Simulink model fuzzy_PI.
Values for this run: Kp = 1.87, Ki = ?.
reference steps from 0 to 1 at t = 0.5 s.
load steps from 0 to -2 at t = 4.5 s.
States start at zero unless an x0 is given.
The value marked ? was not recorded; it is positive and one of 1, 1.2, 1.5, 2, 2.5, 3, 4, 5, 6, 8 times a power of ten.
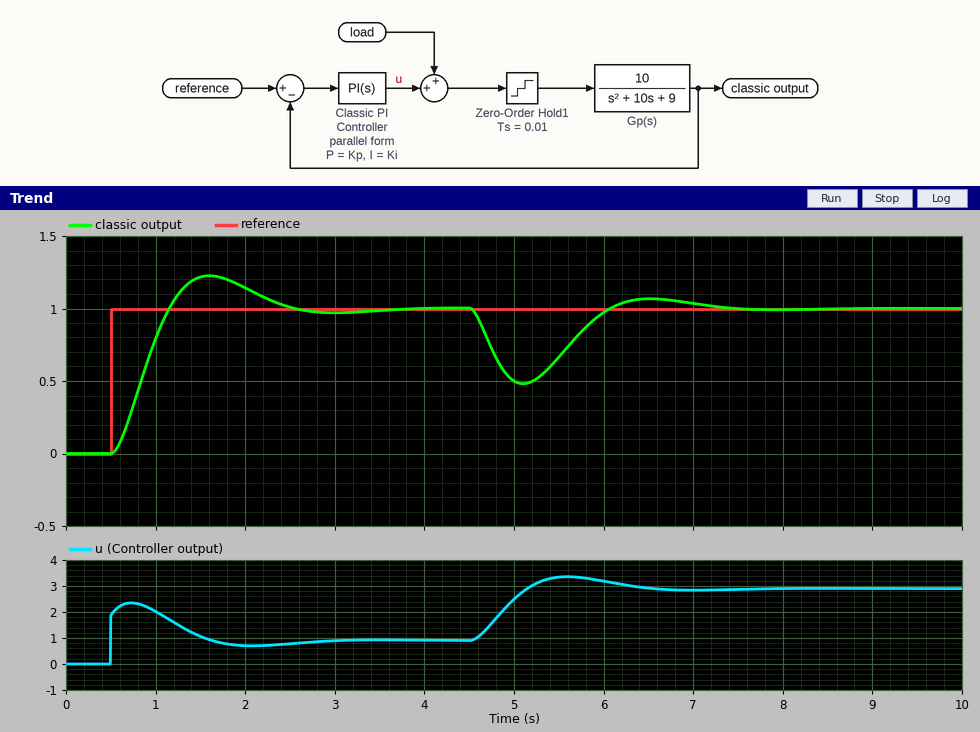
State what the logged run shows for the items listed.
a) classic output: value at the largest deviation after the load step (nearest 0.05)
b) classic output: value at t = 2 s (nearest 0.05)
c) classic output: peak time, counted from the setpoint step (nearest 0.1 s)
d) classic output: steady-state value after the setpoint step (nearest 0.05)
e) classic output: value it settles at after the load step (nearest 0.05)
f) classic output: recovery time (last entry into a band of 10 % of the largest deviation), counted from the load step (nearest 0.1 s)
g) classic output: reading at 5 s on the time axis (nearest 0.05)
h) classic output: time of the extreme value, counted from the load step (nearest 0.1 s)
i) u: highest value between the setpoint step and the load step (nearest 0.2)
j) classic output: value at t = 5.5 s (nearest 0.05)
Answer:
0.50
1.15
1.1 s
1.00
1.00
2.3 s
0.50
0.6 s
2.4
0.65
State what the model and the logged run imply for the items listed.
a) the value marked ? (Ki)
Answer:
5
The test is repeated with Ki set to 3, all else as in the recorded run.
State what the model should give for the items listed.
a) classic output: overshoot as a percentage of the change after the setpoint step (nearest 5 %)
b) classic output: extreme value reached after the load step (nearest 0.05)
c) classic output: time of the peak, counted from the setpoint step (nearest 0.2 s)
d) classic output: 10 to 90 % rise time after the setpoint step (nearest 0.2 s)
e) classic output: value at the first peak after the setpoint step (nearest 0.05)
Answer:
10 %
0.45
1.4 s
0.6 s
1.10
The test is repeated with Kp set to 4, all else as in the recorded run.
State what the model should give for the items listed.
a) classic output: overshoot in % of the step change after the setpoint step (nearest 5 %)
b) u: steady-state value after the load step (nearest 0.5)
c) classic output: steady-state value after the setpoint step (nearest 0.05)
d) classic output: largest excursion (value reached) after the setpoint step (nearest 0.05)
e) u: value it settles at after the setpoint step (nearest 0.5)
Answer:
10 %
3.0
1.00
1.10
1.0
